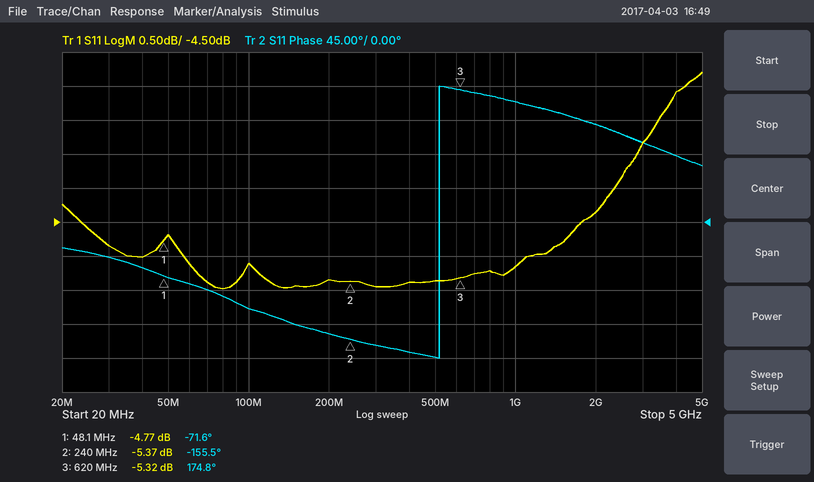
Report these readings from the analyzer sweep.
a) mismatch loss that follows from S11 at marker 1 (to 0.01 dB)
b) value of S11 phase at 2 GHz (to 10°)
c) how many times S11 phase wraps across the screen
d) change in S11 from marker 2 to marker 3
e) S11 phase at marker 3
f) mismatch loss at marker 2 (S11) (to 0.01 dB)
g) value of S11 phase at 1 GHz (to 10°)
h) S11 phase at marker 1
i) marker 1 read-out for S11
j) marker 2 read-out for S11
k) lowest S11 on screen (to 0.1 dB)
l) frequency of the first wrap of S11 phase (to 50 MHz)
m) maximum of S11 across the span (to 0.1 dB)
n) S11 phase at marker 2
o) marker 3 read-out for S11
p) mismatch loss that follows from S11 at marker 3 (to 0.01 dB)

1.76 dB
130°
1
0.05 dB
174.8°
1.49 dB
160°
-71.6°
-4.77 dB
-5.37 dB
-5.5 dB
500 MHz
-2.3 dB
-155.5°
-5.32 dB
1.51 dB
